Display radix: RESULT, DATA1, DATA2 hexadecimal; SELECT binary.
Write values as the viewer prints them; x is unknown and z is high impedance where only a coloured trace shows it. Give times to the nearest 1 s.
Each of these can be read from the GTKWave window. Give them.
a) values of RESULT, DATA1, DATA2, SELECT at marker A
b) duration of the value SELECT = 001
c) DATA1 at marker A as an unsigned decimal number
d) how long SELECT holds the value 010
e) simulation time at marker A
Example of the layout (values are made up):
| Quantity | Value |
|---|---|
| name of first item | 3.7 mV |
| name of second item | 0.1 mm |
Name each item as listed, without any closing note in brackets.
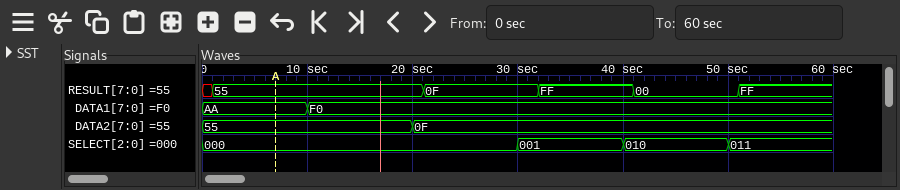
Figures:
| Quantity | Value |
|---|---|
| values of RESULT, DATA1, DATA2, SELECT at marker A | RESULT=55, DATA1=AA, DATA2=55, SELECT=000 |
| duration of the value SELECT = 001 | 10 s |
| DATA1 at marker A as an unsigned decimal number | 170 |
| how long SELECT holds the value 010 | 10 s |
| simulation time at marker A | 7 s |
